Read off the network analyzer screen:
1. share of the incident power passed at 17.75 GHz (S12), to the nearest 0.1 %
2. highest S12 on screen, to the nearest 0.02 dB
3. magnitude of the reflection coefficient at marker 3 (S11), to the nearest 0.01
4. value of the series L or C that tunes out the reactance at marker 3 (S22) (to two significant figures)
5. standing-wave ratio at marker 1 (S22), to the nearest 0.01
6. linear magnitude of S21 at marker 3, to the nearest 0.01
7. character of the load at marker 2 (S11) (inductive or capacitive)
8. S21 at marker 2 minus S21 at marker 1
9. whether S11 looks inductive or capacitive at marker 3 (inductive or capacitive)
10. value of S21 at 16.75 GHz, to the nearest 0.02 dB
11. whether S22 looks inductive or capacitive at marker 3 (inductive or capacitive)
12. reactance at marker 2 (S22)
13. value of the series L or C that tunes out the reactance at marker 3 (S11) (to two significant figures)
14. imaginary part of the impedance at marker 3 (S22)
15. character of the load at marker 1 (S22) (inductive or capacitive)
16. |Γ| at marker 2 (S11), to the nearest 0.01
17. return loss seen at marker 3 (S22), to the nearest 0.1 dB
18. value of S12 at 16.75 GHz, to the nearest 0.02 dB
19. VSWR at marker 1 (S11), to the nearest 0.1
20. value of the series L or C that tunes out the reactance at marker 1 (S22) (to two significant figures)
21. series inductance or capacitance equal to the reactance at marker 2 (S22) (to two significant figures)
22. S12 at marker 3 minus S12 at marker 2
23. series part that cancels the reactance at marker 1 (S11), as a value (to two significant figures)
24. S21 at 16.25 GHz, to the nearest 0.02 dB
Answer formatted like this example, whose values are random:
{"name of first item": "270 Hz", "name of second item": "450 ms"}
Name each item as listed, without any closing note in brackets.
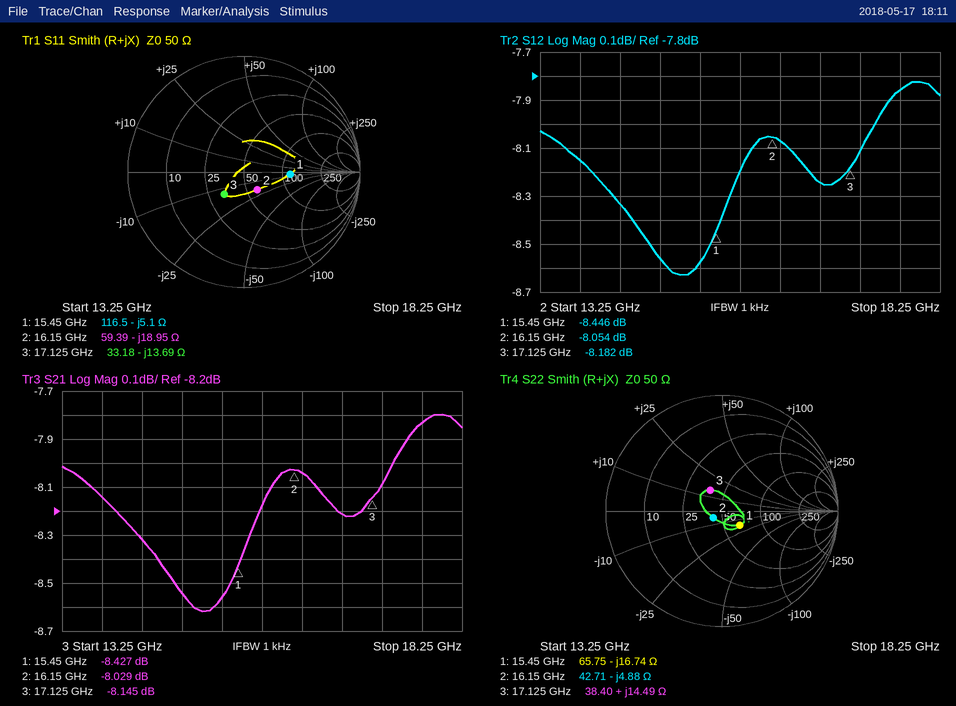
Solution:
{"share of the incident power passed at 17.75 GHz (S12), to the nearest 0.1 %": "16.4 %", "highest S12 on screen, to the nearest 0.02 dB": "-7.82 dB", "magnitude of the reflection coefficient at marker 3 (S11), to the nearest 0.01": "0.26", "value of the series L or C that tunes out the reactance at marker 3 (S22)": "640 fF", "standing-wave ratio at marker 1 (S22), to the nearest 0.01": "1.49", "linear magnitude of S21 at marker 3, to the nearest 0.01": "0.39", "character of the load at marker 2 (S11)": "capacitive", "S21 at marker 2 minus S21 at marker 1": "0.398 dB", "whether S11 looks inductive or capacitive at marker 3": "capacitive", "value of S21 at 16.75 GHz, to the nearest 0.02 dB": "-8.22 dB", "whether S22 looks inductive or capacitive at marker 3": "inductive", "reactance at marker 2": "-4.88 Ω", "value of the series L or C that tunes out the reactance at marker 3 (S11)": "130 pH", "imaginary part of the impedance at marker 3": "+14.49 Ω", "character of the load at marker 1 (S22)": "capacitive", "|Γ| at marker 2 (S11), to the nearest 0.01": "0.19", "return loss seen at marker 3 (S22), to the nearest 0.1 dB": "13.7 dB", "value of S12 at 16.75 GHz, to the nearest 0.02 dB": "-8.24 dB", "VSWR at marker 1 (S11), to the nearest 0.1": "2.3", "value of the series L or C that tunes out the reactance at marker 1 (S22)": "170 pH", "series inductance or capacitance equal to the reactance at marker 2 (S22)": "2.0 pF", "S12 at marker 3 minus S12 at marker 2": "-0.128 dB", "series part that cancels the reactance at marker 1 (S11), as a value": "53 pH", "S21 at 16.25 GHz, to the nearest 0.02 dB": "-8.04 dB"}
